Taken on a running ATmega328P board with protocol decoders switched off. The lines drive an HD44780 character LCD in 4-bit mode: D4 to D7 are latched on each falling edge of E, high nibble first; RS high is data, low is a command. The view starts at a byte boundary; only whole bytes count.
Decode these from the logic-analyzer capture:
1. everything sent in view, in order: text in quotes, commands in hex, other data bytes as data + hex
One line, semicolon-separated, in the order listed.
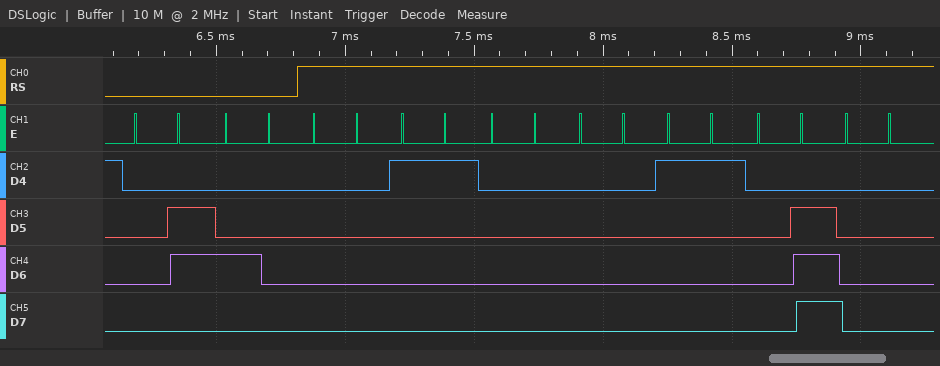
0x06 0x40 data 00 11 00 00 11 0E 00
